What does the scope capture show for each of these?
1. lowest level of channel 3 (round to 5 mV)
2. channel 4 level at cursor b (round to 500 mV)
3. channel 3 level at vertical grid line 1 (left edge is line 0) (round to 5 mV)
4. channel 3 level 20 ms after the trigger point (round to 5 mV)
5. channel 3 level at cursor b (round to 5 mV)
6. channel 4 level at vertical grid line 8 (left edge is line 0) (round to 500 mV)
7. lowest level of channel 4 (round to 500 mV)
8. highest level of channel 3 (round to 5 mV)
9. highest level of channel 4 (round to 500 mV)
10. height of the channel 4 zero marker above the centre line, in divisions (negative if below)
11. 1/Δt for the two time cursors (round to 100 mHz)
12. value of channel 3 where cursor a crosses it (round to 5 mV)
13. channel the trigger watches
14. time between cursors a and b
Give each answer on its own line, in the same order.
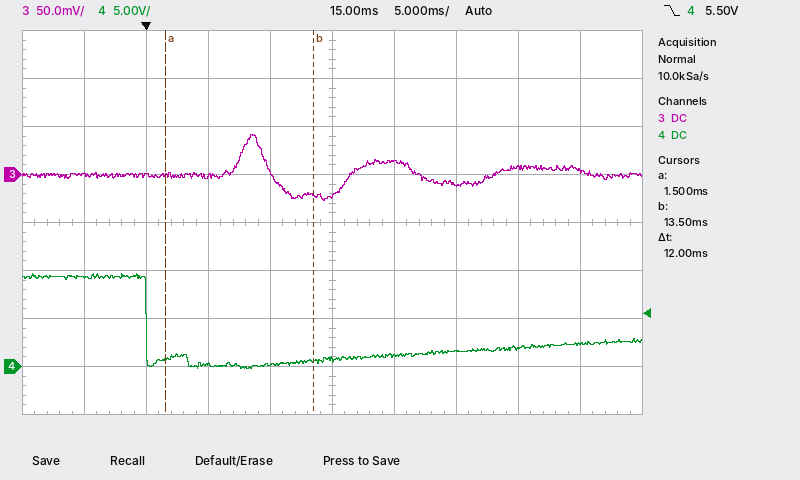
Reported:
-25 mV
500 mV
0 mV
15 mV
-20 mV
2.0 V
0.0 V
40 mV
9.5 V
-3.0 div
83.3 Hz
0 mV
channel 4
12 ms
